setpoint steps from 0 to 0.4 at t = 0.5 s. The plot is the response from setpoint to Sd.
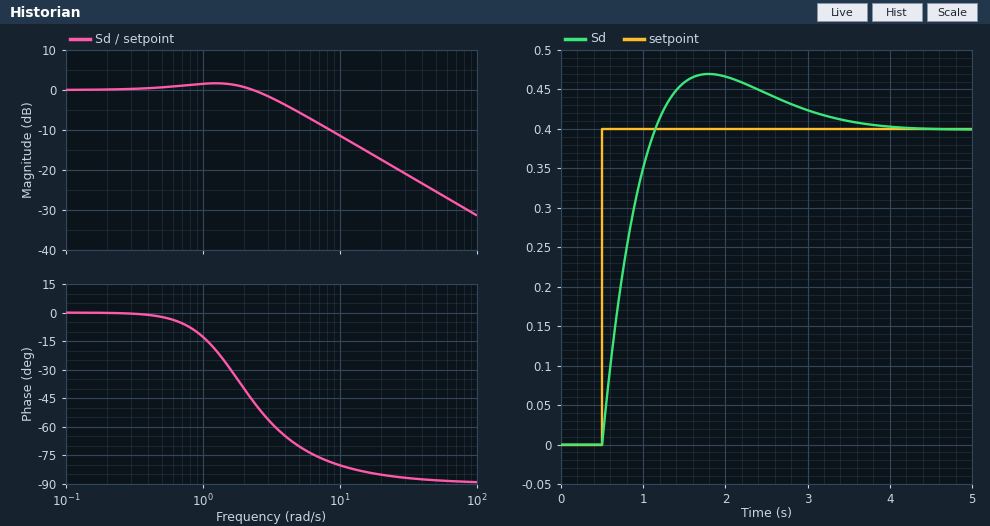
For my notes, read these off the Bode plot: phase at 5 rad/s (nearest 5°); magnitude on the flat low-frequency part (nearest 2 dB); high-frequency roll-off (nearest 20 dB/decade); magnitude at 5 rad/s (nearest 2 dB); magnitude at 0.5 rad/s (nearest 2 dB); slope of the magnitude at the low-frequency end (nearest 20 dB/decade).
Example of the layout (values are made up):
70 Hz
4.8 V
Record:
-70°
0 dB
-20 dB/decade
-6 dB
0 dB
0 dB/decade
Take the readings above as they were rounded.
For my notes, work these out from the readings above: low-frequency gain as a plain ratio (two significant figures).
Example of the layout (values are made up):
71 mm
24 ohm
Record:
1.0
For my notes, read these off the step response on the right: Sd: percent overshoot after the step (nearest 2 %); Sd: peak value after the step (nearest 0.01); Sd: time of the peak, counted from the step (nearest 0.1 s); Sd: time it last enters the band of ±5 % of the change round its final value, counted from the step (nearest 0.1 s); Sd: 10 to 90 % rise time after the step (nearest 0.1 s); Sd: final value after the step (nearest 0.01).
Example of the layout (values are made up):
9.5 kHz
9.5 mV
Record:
18 %
0.47
1.3 s
2.6 s
0.5 s
0.40
